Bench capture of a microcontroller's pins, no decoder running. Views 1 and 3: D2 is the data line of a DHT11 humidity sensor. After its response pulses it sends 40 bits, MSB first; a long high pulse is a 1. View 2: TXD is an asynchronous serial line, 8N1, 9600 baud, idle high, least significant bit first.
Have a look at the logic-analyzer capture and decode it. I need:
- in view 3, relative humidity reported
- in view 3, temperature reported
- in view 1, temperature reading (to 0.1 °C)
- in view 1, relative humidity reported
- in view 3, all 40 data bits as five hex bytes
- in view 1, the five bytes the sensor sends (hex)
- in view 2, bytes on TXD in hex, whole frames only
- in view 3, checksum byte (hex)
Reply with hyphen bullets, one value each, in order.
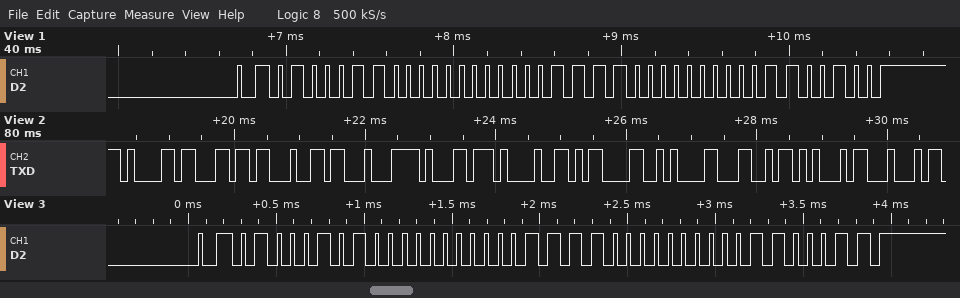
- 69 %
- 30.0 °C
- 30.0 °C
- 70 %
- 45 00 1E 00 63
- 46 00 1E 00 64
- 61 6C 64 C4 B1 21 0D 0A 4C 45 44
- 0x63
